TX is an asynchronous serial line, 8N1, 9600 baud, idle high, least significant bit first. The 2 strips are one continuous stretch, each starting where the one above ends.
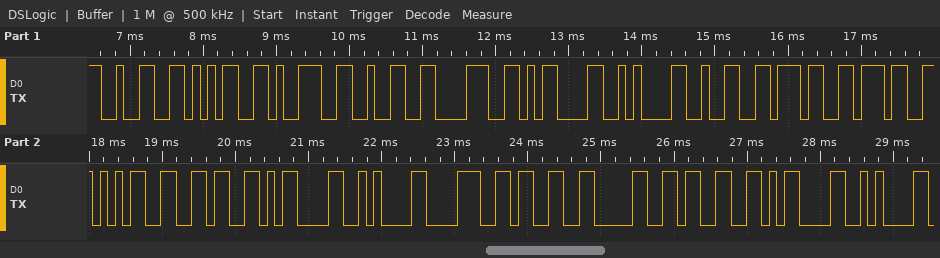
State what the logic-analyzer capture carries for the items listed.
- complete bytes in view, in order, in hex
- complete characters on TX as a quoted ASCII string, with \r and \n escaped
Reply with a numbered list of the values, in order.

1. 32 35 39 32 38 0D 0A 32 37 37 35 36 0D 0A 38 33 30 33 0D 0A
2. "25928\r\n27756\r\n8303\r\n"
